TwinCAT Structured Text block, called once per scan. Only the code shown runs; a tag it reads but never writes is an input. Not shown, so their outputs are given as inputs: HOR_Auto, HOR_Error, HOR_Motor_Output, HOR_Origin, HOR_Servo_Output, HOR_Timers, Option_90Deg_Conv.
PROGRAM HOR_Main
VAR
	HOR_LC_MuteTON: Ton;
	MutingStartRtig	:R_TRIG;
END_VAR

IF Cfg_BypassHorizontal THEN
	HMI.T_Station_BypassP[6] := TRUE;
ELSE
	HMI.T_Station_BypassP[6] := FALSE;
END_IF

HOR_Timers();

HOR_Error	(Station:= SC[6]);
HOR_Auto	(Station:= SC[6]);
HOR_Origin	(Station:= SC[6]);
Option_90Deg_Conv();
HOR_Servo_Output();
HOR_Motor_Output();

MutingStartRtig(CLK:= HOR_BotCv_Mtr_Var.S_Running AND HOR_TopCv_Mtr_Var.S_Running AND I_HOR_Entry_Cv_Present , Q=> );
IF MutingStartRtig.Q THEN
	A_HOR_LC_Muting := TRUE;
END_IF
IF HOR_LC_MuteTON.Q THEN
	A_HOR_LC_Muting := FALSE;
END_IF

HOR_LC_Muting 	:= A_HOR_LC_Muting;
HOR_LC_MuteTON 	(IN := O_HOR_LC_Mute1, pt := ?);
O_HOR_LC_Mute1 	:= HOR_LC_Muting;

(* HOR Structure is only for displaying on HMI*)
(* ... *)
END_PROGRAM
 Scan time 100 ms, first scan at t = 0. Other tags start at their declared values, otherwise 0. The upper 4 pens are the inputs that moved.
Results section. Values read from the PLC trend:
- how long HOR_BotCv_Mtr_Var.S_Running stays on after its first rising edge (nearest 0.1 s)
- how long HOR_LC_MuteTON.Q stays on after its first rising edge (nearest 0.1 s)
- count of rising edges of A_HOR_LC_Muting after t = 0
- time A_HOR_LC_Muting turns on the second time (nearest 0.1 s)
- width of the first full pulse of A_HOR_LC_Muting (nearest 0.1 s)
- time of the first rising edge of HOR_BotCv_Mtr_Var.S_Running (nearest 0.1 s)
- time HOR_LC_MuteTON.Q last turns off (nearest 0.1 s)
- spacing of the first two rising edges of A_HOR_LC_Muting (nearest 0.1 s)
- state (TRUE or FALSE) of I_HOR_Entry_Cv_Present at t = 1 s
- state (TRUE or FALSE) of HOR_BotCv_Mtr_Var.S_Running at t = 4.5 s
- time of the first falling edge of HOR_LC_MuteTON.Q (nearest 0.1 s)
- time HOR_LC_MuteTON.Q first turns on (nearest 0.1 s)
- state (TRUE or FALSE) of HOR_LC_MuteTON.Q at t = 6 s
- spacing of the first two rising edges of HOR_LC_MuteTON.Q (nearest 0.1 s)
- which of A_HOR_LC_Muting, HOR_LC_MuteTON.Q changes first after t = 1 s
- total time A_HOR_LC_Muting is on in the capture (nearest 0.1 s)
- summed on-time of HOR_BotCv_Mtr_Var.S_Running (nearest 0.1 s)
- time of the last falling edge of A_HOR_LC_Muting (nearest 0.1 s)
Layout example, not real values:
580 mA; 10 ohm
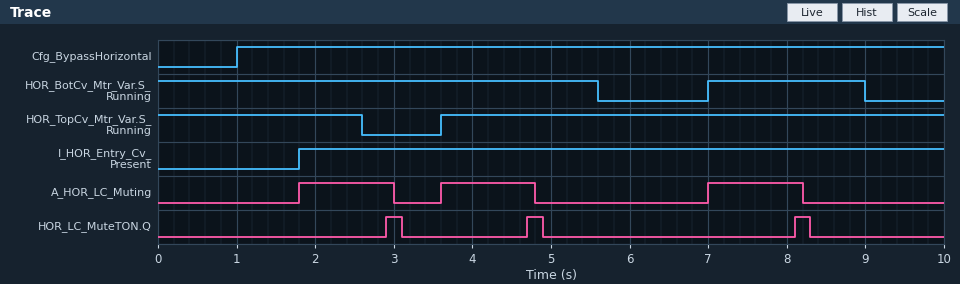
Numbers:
2.0 s; 0.2 s; 3; 3.6 s; 1.2 s; 7.0 s; 8.3 s; 1.8 s; FALSE; TRUE; 3.1 s; 2.9 s; FALSE; 1.8 s; A_HOR_LC_Muting; 3.6 s; 7.6 s; 8.2 s
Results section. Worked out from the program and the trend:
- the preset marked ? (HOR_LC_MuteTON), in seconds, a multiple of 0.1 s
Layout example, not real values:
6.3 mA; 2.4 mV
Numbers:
1.0 s
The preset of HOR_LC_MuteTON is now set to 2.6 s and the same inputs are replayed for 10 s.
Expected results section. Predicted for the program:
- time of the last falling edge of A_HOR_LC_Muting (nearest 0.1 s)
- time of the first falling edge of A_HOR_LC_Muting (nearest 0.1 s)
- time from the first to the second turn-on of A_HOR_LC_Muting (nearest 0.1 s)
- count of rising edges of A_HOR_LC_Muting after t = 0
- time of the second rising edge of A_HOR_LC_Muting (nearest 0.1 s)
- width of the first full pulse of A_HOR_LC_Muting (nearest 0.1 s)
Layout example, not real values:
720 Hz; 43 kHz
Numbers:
9.8 s; 4.6 s; 5.2 s; 2; 7.0 s; 2.8 s
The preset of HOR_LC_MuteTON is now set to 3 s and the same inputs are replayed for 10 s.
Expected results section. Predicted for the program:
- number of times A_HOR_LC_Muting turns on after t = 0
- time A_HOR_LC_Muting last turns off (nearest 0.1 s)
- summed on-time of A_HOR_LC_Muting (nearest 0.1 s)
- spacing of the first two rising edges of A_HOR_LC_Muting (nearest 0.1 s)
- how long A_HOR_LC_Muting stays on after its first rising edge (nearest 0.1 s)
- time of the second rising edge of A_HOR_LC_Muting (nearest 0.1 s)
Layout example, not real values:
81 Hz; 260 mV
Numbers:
2; 5.0 s; 6.2 s; 5.2 s; 3.2 s; 7.0 s
